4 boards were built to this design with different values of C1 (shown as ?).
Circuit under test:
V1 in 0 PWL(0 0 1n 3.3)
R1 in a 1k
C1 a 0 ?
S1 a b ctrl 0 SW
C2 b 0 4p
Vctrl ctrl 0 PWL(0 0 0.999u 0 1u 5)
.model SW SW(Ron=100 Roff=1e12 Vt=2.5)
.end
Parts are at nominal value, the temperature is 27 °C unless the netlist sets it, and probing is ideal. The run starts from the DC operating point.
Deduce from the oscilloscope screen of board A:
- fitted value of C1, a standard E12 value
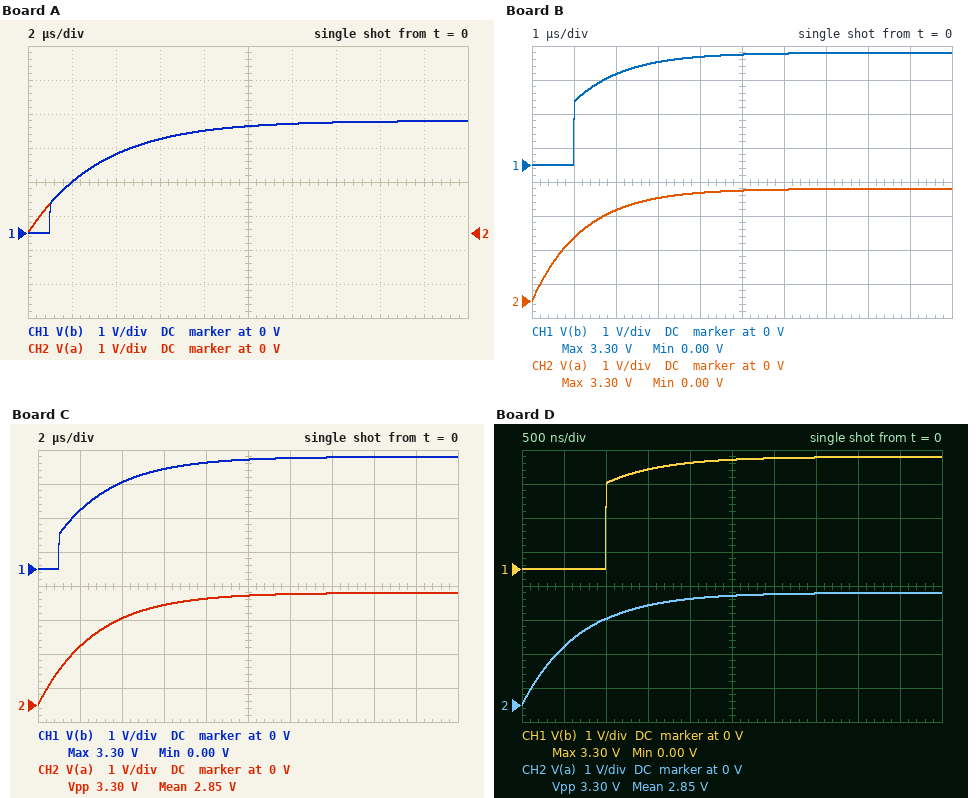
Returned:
3.3 nF
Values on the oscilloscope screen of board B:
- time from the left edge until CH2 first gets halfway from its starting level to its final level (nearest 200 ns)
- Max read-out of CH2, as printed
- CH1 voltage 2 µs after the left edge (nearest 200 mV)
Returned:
800 ns
3.30 V
2.6 V
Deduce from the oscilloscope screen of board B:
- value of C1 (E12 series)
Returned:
1.2 nF
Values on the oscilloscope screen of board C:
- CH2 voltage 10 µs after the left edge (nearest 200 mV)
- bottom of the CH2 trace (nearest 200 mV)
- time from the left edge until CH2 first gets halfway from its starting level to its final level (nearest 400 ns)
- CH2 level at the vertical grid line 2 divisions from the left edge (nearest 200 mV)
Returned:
3.2 V
0 V
2.0 µs
2.6 V
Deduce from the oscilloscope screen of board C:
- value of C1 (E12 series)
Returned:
2.7 nF
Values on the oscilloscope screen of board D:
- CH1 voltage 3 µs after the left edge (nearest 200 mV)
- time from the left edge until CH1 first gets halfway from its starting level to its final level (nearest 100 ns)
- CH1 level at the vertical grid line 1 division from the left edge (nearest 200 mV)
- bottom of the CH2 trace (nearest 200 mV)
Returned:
3.2 V
1.0 µs
0 V
0 V
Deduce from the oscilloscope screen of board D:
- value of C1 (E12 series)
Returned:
680 pF
